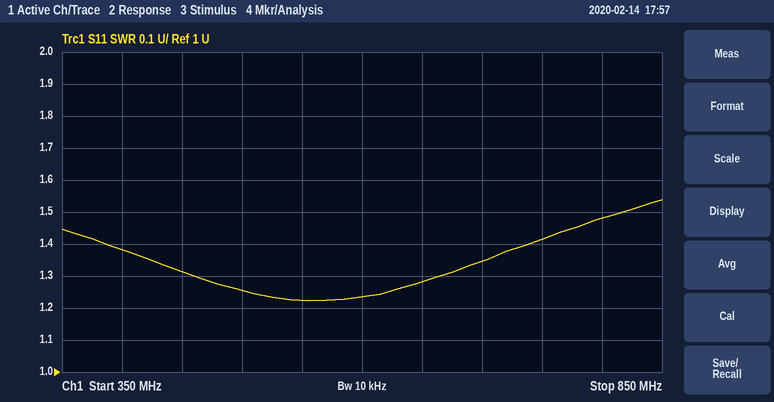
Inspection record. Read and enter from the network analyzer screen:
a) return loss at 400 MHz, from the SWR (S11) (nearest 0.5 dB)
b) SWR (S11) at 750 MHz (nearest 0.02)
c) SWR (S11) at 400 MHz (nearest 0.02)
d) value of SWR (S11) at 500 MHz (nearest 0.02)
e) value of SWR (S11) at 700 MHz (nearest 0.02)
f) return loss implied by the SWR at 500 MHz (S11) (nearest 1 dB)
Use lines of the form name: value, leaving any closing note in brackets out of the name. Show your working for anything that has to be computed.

return loss at 400 MHz, from the SWR (S11): −20 log10((1.38 − 1)/(1.38 + 1)) ≈ 15.9 dB, so 16.0 dB to the nearest 0.5 dB
SWR (S11) at 750 MHz: 1.42
SWR (S11) at 400 MHz: 1.38
value of SWR (S11) at 500 MHz: 1.26
value of SWR (S11) at 700 MHz: 1.34
return loss implied by the SWR at 500 MHz (S11): −20 log10((1.26 − 1)/(1.26 + 1)) ≈ 19 dB
